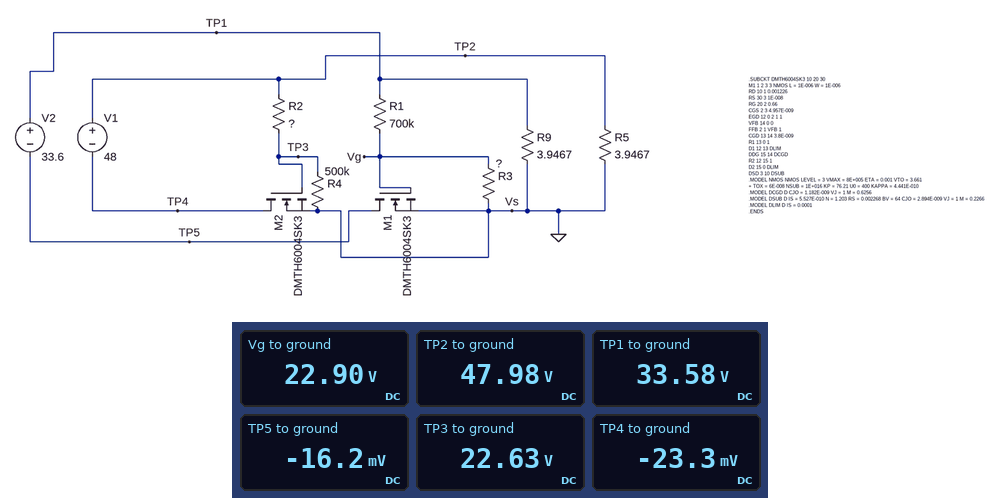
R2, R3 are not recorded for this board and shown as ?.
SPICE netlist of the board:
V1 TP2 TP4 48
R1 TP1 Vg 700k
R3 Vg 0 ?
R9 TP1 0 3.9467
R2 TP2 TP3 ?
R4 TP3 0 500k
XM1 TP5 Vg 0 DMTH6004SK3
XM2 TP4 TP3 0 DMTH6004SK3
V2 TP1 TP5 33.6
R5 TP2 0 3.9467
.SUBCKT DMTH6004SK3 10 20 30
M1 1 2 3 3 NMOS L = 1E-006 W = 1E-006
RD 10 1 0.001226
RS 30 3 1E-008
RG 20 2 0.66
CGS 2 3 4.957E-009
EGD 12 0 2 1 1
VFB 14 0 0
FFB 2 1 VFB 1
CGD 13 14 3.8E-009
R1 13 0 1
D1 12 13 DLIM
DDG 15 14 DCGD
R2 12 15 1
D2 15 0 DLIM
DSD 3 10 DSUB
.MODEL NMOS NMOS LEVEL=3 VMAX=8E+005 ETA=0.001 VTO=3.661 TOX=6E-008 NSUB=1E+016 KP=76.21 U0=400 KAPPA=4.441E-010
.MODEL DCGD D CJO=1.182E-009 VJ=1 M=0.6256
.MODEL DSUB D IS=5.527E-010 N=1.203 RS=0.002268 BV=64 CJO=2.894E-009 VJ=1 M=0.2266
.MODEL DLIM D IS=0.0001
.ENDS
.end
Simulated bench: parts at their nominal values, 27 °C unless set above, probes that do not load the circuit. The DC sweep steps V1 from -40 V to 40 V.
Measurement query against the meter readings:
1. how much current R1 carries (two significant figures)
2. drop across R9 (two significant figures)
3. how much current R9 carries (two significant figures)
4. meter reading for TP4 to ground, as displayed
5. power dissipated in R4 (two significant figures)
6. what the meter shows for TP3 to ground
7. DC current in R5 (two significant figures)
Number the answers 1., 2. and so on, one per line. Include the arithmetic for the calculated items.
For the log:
1. (33.58 V - 22.9 V) / 700 kΩ = 15 µA
2. 33.58 V = 34 V
3. (33.58 V) / 3.947 Ω = 8.5 A
4. -23.3 mV
5. (22.63 V)^2 / 500 kΩ = 1.0 mW
6. 22.63 V
7. (47.98 V) / 3.947 Ω = 12 A
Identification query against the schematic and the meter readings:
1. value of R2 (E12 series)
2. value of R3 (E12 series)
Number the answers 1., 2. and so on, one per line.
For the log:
1. 560 kΩ
2. 1.5 MΩ
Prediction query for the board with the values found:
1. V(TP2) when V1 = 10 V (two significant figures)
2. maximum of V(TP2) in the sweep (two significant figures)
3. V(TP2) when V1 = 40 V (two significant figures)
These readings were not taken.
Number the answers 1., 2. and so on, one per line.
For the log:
1. 10 V
2. 40 V
3. 40 V
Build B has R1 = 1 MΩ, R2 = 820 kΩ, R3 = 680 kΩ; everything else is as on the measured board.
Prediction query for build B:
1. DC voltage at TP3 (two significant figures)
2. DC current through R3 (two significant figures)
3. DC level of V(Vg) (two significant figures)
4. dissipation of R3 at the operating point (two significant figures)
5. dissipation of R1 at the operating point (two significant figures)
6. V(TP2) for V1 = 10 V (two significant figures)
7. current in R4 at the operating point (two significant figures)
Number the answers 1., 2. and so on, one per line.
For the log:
1. 18 V
2. 20 µA
3. 14 V
4. 270 µW
5. 400 µW
6. 9.8 V
7. 36 µA
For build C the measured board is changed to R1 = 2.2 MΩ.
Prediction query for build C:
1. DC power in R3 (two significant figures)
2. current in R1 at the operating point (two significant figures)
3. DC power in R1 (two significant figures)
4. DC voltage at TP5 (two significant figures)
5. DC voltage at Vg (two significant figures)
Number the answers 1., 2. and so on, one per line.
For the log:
1. 120 µW
2. 9.1 µA
3. 180 µW
4. -22 mV
5. 14 V
